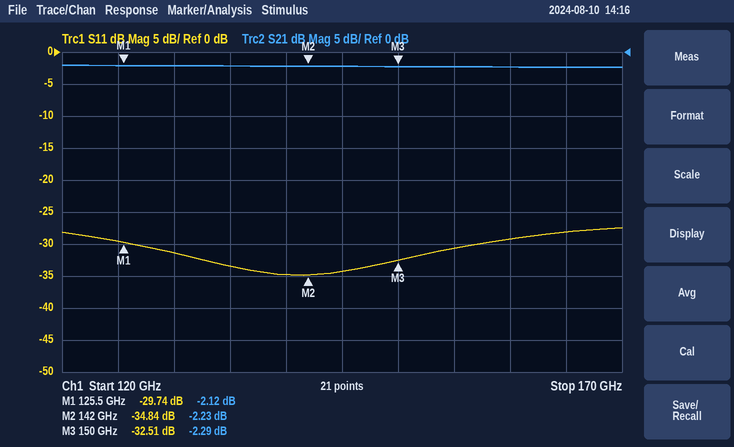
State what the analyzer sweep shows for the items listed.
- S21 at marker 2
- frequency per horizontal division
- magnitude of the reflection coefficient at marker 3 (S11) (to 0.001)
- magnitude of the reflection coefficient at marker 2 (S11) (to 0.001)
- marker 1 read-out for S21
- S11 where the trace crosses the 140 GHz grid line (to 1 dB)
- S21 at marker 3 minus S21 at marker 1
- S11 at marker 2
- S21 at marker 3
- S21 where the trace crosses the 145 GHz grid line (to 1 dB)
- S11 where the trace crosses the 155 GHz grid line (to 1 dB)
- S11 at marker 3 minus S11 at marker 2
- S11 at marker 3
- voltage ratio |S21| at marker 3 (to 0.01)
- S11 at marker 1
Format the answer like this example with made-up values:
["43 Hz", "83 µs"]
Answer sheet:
["-2.23 dB", "5 GHz", "0.024", "0.018", "-2.12 dB", "-35 dB", "-0.17 dB", "-34.84 dB", "-2.29 dB", "-2 dB", "-31 dB", "2.33 dB", "-32.51 dB", "0.77", "-29.74 dB"]
